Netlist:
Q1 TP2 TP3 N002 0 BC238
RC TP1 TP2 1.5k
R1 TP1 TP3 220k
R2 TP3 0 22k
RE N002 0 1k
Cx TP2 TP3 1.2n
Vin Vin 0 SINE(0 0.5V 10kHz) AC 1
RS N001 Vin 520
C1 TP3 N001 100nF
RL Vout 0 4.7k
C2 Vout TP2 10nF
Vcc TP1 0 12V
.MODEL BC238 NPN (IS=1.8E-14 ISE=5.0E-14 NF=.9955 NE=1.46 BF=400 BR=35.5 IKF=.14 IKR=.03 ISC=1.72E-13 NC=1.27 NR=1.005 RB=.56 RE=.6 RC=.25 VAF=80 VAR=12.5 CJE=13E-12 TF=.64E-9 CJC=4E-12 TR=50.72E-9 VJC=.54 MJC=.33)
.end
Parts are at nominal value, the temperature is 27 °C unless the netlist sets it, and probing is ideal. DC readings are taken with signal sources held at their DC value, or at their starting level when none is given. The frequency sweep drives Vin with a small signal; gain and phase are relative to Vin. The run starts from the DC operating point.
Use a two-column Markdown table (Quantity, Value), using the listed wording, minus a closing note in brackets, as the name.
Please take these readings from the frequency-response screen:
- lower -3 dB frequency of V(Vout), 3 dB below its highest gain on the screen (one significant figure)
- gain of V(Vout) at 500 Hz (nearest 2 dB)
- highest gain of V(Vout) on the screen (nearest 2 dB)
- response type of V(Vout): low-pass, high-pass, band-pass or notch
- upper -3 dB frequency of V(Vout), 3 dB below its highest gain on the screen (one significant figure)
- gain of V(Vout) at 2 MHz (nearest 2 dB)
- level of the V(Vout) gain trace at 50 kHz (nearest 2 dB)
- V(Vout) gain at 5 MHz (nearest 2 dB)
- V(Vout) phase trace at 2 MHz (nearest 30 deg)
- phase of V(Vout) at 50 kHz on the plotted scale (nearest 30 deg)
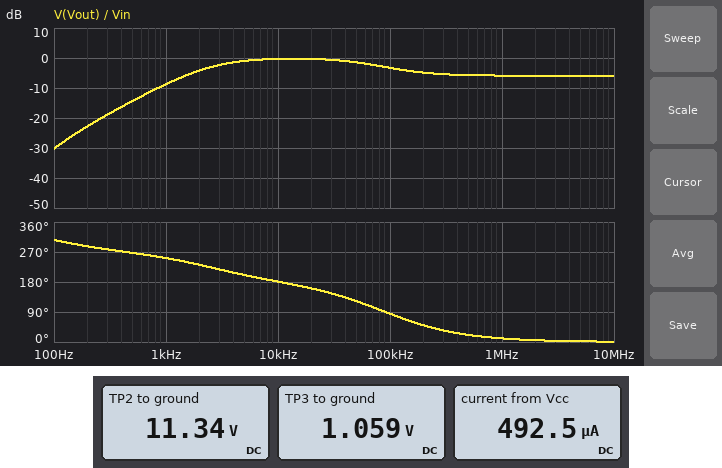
| Quantity | Value |
|---|---|
| lower -3 dB frequency of V(Vout), 3 dB below its highest gain on the screen | 2 kHz |
| gain of V(Vout) at 500 Hz | -14 dB |
| highest gain of V(Vout) on the screen | 0 dB |
| response type of V(Vout): low-pass, high-pass, band-pass or notch | high-pass |
| upper -3 dB frequency of V(Vout), 3 dB below its highest gain on the screen | 100 kHz |
| gain of V(Vout) at 2 MHz | -6 dB |
| level of the V(Vout) gain trace at 50 kHz | -2 dB |
| V(Vout) gain at 5 MHz | -6 dB |
| V(Vout) phase trace at 2 MHz | 0 deg |
| phase of V(Vout) at 50 kHz on the plotted scale | 120 deg |
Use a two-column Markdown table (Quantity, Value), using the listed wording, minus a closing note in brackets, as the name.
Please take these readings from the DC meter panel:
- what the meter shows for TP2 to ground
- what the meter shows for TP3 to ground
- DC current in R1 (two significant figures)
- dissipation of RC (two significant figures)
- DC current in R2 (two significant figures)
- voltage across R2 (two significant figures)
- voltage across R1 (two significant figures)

| Quantity | Value |
|---|---|
| what the meter shows for TP2 to ground | 11.34 V |
| what the meter shows for TP3 to ground | 1.059 V |
| DC current in R1 | 50 µA |
| dissipation of RC | 290 µW |
| DC current in R2 | 48 µA |
| voltage across R2 | 1.1 V |
| voltage across R1 | 11 V |
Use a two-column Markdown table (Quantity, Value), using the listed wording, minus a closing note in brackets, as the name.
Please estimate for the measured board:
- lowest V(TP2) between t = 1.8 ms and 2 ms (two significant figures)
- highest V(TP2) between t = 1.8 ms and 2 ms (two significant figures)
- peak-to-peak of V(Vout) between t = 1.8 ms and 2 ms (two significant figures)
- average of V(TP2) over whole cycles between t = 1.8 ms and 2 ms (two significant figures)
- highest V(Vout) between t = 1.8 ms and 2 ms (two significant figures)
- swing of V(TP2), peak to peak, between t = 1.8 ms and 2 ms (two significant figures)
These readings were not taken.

| Quantity | Value |
|---|---|
| lowest V(TP2) between t = 1.8 ms and 2 ms | 11 V |
| highest V(TP2) between t = 1.8 ms and 2 ms | 12 V |
| peak-to-peak of V(Vout) between t = 1.8 ms and 2 ms | 940 mV |
| average of V(TP2) over whole cycles between t = 1.8 ms and 2 ms | 11 V |
| highest V(Vout) between t = 1.8 ms and 2 ms | 460 mV |
| swing of V(TP2), peak to peak, between t = 1.8 ms and 2 ms | 990 mV |
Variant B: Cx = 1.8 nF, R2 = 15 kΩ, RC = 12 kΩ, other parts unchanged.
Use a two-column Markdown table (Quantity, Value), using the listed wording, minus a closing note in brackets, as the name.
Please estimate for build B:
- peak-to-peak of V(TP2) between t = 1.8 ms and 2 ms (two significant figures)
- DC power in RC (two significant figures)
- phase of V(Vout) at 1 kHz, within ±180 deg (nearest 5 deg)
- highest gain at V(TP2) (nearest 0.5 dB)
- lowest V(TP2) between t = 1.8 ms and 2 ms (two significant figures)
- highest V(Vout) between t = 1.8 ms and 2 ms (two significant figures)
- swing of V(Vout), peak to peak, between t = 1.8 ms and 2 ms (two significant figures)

| Quantity | Value |
|---|---|
| peak-to-peak of V(TP2) between t = 1.8 ms and 2 ms | 1.9 V |
| DC power in RC | 330 µW |
| phase of V(Vout) at 1 kHz, within ±180 deg | -135 deg |
| highest gain at V(TP2) | 17.5 dB |
| lowest V(TP2) between t = 1.8 ms and 2 ms | 8.4 V |
| highest V(Vout) between t = 1.8 ms and 2 ms | 730 mV |
| swing of V(Vout), peak to peak, between t = 1.8 ms and 2 ms | 1.7 V |
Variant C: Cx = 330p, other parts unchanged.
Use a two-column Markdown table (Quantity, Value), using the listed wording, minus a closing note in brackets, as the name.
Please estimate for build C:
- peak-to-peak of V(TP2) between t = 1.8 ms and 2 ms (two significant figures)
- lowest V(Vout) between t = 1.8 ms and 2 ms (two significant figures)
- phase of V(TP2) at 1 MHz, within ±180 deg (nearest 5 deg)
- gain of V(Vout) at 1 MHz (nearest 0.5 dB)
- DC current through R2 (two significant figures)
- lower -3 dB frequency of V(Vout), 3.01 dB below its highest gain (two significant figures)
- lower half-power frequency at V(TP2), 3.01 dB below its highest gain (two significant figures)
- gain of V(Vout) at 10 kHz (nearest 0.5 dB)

| Quantity | Value |
|---|---|
| peak-to-peak of V(TP2) between t = 1.8 ms and 2 ms | 1.0 V |
| lowest V(Vout) between t = 1.8 ms and 2 ms | -500 mV |
| phase of V(TP2) at 1 MHz, within ±180 deg | 35 deg |
| gain of V(Vout) at 1 MHz | -5.5 dB |
| DC current through R2 | 48 µA |
| lower -3 dB frequency of V(Vout), 3.01 dB below its highest gain | 2.5 kHz |
| lower half-power frequency at V(TP2), 3.01 dB below its highest gain | 78 Hz |
| gain of V(Vout) at 10 kHz | 0 dB |
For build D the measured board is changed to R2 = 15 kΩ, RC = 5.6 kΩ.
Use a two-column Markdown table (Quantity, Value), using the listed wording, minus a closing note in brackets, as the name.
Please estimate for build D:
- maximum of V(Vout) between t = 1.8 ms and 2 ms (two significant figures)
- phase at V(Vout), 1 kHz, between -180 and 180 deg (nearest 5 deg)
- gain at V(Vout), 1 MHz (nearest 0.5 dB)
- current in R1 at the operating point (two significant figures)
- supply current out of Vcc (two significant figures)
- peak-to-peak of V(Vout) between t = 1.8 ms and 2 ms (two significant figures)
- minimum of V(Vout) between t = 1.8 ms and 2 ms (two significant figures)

| Quantity | Value |
|---|---|
| maximum of V(Vout) between t = 1.8 ms and 2 ms | 560 mV |
| phase at V(Vout), 1 kHz, between -180 and 180 deg | -120 deg |
| gain at V(Vout), 1 MHz | -4.5 dB |
| current in R1 at the operating point | 51 µA |
| supply current out of Vcc | 220 µA |
| peak-to-peak of V(Vout) between t = 1.8 ms and 2 ms | 1.4 V |
| minimum of V(Vout) between t = 1.8 ms and 2 ms | -840 mV |
